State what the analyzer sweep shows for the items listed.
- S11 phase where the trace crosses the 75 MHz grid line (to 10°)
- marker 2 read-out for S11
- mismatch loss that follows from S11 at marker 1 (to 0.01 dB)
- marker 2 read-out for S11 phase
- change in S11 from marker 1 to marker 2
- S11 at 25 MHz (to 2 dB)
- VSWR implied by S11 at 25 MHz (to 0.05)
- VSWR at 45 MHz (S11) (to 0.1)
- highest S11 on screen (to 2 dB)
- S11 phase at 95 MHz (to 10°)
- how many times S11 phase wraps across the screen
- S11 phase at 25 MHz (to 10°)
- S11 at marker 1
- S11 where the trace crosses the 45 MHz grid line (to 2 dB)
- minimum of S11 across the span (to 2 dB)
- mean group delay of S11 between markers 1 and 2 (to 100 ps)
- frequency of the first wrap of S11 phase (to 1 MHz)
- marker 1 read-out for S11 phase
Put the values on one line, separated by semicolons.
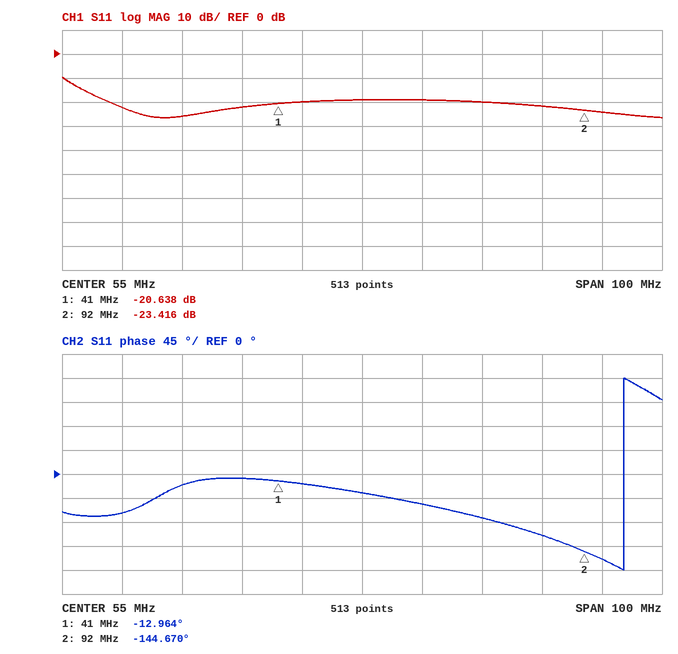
-80°; -23.416 dB; 0.04 dB; -144.670°; -2.778 dB; -26 dB; 1.10; 1.2; -10 dB; -160°; 1; -20°; -20.638 dB; -20 dB; -26 dB; 7.2 ns; 99 MHz; -12.964°
